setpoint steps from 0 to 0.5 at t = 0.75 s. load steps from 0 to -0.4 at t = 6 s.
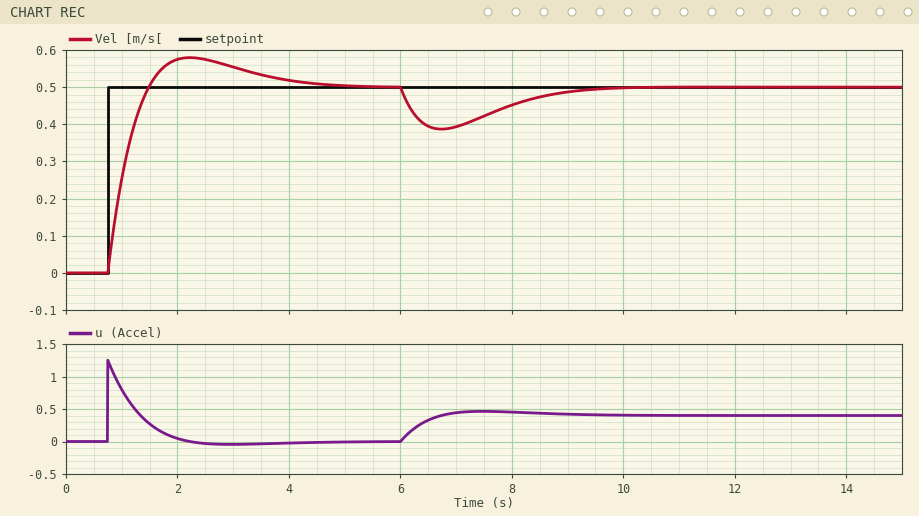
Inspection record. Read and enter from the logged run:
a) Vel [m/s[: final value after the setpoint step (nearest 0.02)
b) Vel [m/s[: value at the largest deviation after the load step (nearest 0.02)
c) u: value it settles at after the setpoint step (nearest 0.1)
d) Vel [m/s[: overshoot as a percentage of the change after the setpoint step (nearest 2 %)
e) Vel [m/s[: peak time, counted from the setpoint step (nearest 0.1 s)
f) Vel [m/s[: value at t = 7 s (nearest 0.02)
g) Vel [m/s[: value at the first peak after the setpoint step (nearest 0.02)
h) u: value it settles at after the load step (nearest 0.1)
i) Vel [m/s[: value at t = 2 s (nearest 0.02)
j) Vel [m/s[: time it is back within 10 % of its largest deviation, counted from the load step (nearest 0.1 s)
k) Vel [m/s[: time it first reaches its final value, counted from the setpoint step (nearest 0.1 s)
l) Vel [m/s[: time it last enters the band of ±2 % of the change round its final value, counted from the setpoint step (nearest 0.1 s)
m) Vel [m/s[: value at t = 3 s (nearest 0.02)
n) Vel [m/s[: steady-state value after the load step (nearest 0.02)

0.50
0.38
0.0
16 %
1.5 s
0.40
0.58
0.4
0.58
3.1 s
0.7 s
3.7 s
0.56
0.50
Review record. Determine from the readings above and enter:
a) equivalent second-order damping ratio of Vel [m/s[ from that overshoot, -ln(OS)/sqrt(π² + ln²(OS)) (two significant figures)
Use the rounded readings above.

0.50
